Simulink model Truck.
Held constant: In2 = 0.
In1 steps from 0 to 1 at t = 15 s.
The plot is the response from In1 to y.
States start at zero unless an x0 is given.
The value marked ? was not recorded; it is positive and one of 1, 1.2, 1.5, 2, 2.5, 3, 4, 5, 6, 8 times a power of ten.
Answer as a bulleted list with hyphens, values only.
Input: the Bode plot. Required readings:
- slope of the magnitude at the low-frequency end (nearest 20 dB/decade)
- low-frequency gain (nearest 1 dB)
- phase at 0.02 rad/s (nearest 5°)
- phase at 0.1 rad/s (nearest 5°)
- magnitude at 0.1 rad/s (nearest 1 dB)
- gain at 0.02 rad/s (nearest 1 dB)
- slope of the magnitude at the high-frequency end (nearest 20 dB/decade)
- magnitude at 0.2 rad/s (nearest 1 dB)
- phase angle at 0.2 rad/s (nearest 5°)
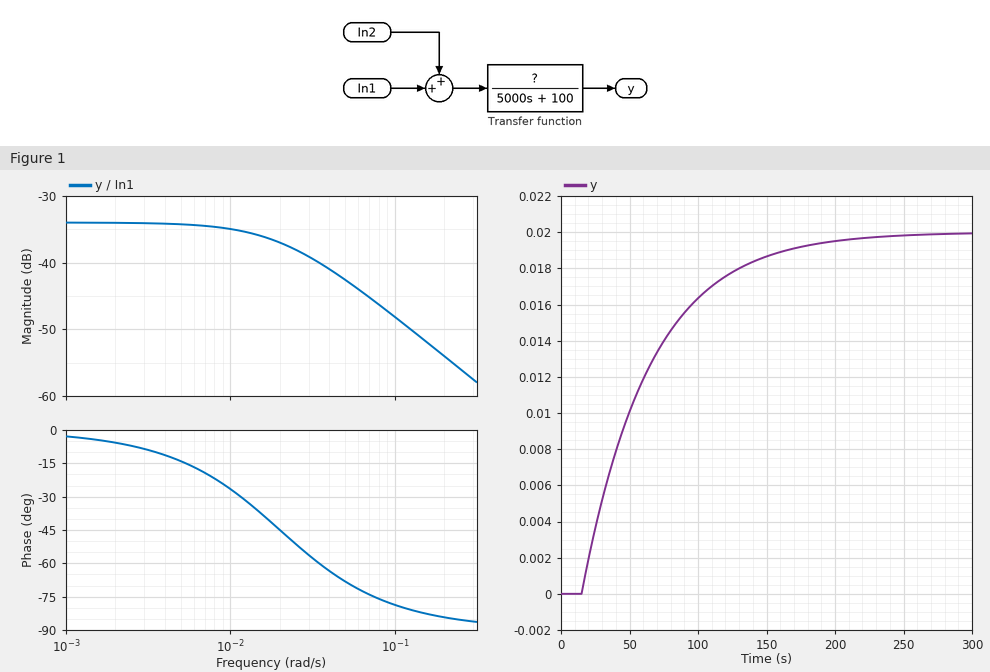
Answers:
- 0 dB/decade
- -34 dB
- -45°
- -80°
- -48 dB
- -37 dB
- -20 dB/decade
- -54 dB
- -85°
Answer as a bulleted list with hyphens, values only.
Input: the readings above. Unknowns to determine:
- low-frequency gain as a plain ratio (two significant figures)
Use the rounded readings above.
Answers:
- 0.020
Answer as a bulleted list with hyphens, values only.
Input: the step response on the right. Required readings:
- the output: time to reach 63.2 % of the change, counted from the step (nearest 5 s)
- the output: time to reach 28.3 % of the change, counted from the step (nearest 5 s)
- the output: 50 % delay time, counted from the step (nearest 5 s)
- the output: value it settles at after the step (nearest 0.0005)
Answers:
- 50 s
- 15 s
- 35 s
- 0.0200
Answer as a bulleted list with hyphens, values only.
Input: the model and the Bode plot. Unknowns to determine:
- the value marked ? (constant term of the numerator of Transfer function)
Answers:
- 2
